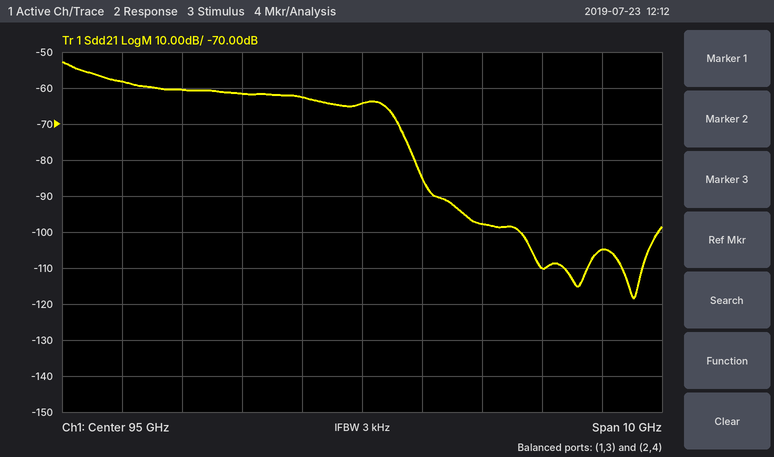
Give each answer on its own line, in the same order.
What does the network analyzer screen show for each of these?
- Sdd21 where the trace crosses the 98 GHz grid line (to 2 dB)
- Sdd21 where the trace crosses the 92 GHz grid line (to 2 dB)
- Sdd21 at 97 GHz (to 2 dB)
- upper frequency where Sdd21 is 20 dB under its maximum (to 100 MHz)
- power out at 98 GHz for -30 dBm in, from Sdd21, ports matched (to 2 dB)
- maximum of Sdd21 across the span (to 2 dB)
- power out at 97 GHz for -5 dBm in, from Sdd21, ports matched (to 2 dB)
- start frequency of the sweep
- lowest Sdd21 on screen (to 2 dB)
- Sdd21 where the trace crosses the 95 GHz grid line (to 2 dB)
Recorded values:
-110 dB
-60 dB
-98 dB
95.7 GHz
-140 dBm
-52 dB
-102 dBm
90 GHz
-118 dB
-64 dB
